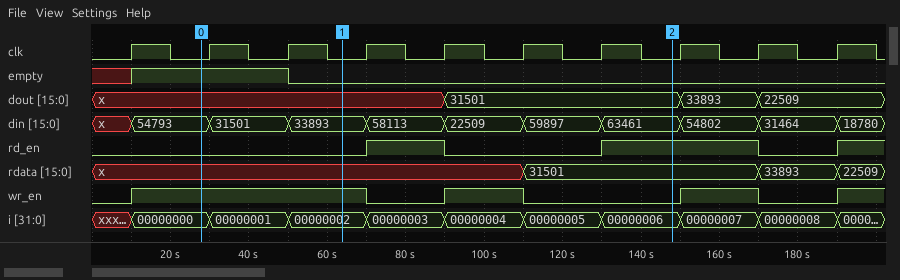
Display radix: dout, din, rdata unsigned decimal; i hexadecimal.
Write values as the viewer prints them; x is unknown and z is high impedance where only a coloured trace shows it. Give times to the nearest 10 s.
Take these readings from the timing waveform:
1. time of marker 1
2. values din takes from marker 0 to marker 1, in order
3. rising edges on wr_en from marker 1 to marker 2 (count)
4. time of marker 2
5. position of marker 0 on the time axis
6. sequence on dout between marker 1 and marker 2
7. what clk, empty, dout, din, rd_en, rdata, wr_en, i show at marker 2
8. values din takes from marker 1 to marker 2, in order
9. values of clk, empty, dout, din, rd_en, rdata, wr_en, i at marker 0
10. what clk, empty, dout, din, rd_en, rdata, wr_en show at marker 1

60 s
54793, 31501, 33893
1
150 s
30 s
x, 31501
clk=0, empty=0, dout=31501, din=63461, rd_en=1, rdata=31501, wr_en=0, i=00000006
33893, 58113, 22509, 59897, 63461
clk=0, empty=1, dout=x, din=54793, rd_en=0, rdata=x, wr_en=1, i=00000000
clk=0, empty=0, dout=x, din=33893, rd_en=0, rdata=x, wr_en=1
